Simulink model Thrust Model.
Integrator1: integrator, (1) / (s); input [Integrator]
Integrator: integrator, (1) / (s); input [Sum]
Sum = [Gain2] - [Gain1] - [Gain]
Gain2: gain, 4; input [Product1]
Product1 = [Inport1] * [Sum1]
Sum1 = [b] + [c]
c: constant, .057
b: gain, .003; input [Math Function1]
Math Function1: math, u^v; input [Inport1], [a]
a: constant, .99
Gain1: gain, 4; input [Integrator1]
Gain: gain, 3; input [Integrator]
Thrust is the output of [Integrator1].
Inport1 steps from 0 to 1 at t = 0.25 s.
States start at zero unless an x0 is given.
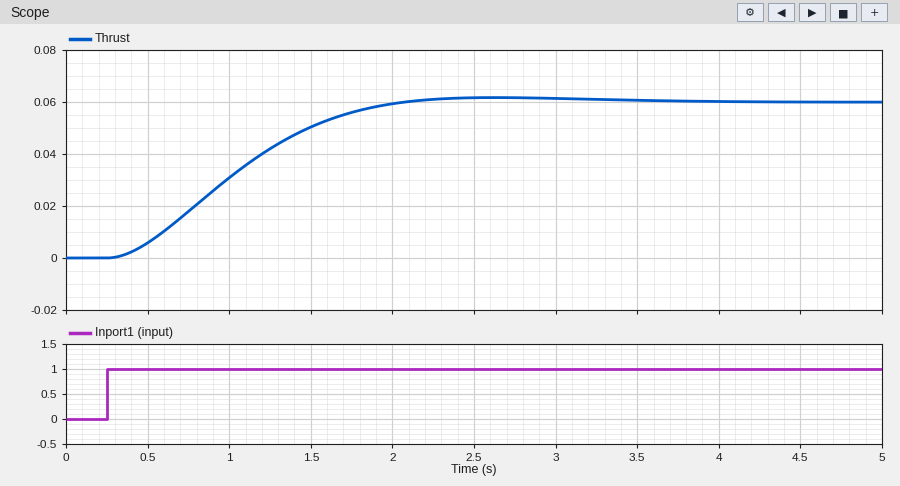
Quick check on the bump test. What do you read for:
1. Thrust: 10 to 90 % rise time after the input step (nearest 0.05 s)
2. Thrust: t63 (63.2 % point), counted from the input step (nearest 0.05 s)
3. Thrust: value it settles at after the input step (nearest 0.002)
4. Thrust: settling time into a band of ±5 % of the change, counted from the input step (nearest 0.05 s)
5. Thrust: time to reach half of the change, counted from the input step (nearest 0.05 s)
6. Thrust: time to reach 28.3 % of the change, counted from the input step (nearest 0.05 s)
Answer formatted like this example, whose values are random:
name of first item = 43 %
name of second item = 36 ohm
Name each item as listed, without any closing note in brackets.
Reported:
Thrust: 10 to 90 % rise time after the input step = 1.15 s
Thrust: t63 (63.2 % point), counted from the input step = 0.90 s
Thrust: value it settles at after the input step = 0.060
Thrust: settling time into a band of ±5 % of the change, counted from the input step = 1.55 s
Thrust: time to reach half of the change, counted from the input step = 0.75 s
Thrust: time to reach 28.3 % of the change, counted from the input step = 0.50 s
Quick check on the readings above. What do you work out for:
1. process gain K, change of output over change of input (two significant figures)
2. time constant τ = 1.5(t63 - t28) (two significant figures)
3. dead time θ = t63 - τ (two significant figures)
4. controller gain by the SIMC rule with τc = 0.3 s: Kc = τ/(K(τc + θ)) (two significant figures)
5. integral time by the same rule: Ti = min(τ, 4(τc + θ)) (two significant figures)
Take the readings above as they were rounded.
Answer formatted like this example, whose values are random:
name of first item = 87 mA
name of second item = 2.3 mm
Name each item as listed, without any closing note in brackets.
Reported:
process gain K, change of output over change of input = 0.060
time constant τ = 1.5(t63 - t28) = 0.60 s
dead time θ = t63 - τ = 0.30 s
controller gain by the SIMC rule with τc = 0.3 s: Kc = τ/(K(τc + θ)) = 17
integral time by the same rule: Ti = min(τ, 4(τc + θ)) = 0.60 s
